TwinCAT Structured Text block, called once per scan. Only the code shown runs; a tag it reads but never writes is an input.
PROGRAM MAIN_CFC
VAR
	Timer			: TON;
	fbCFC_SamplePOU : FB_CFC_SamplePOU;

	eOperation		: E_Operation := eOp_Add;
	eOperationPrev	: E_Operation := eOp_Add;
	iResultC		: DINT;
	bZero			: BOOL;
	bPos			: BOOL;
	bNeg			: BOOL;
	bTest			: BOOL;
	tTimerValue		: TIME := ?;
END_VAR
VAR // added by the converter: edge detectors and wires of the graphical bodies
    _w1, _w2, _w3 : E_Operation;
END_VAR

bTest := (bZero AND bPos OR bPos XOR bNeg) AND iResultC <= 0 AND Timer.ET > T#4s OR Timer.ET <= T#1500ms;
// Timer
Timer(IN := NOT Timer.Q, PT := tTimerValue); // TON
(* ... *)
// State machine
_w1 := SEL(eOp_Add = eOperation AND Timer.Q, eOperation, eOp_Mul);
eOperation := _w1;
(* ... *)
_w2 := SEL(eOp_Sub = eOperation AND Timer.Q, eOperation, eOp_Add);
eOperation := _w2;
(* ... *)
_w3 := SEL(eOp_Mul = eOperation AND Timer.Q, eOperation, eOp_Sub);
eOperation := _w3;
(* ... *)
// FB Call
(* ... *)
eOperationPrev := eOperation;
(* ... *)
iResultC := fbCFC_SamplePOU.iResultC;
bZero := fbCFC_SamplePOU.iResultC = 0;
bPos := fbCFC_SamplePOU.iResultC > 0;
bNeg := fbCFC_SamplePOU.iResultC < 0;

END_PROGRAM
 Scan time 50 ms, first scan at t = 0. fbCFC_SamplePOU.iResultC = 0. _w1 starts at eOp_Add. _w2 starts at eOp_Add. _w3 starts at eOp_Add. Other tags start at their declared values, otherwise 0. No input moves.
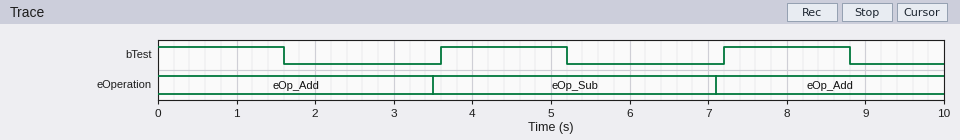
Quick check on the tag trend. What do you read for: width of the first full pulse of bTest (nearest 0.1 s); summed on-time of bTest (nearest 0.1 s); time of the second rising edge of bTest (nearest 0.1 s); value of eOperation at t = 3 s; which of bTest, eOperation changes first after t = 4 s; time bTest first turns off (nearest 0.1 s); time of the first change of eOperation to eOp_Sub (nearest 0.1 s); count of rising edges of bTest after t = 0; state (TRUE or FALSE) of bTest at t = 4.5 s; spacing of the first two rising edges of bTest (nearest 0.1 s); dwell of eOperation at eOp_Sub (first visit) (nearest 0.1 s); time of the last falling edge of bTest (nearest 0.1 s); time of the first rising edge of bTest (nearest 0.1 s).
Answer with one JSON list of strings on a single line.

["1.6 s", "4.8 s", "7.2 s", "eOp_Add", "bTest", "1.6 s", "3.5 s", "2", "TRUE", "3.6 s", "3.6 s", "8.8 s", "3.6 s"]
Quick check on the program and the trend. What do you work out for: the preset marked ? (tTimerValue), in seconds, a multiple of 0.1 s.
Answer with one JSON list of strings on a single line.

["3.5 s"]
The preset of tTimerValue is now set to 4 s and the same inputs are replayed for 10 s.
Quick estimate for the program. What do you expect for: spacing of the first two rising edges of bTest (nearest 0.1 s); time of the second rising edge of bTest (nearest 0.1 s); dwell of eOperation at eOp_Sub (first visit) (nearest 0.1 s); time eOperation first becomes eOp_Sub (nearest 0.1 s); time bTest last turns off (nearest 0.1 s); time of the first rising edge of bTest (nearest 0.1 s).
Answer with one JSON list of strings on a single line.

["4.1 s", "8.2 s", "4.1 s", "4.0 s", "9.8 s", "4.1 s"]
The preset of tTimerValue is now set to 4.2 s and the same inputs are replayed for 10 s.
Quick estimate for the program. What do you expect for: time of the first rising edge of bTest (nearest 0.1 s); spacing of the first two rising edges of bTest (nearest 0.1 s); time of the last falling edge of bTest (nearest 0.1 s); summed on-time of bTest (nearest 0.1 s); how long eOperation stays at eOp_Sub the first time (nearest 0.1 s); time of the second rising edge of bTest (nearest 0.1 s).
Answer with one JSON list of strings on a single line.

["4.3 s", "4.3 s", "5.9 s", "4.6 s", "4.3 s", "8.6 s"]
